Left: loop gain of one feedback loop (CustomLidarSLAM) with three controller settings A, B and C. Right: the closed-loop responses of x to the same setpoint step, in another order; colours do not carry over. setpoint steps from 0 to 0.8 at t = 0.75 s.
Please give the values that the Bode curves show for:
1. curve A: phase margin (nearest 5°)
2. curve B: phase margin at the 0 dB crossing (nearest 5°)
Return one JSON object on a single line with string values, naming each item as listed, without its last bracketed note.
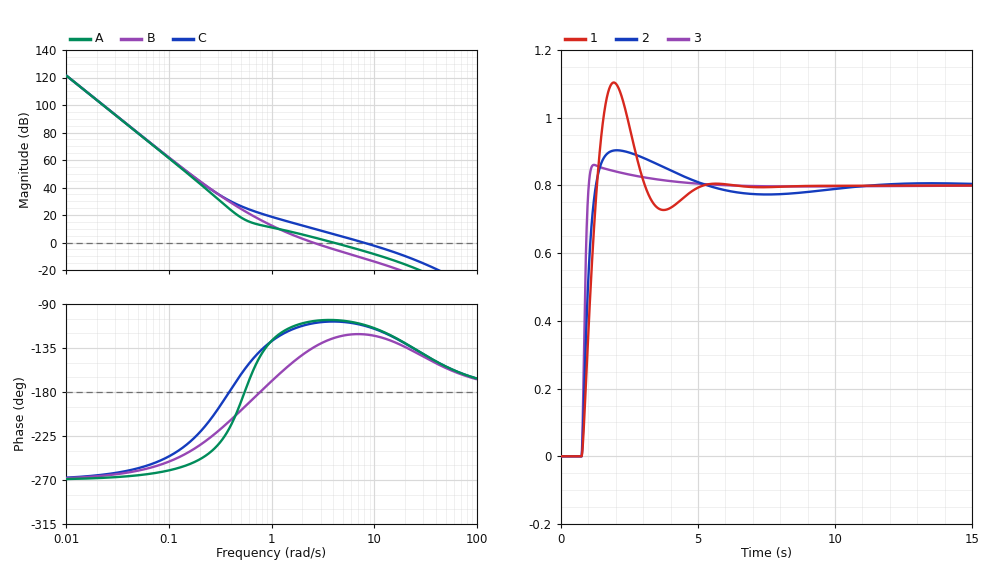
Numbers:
{"curve A: phase margin": "75°", "curve B: phase margin at the 0 dB crossing": "45°"}
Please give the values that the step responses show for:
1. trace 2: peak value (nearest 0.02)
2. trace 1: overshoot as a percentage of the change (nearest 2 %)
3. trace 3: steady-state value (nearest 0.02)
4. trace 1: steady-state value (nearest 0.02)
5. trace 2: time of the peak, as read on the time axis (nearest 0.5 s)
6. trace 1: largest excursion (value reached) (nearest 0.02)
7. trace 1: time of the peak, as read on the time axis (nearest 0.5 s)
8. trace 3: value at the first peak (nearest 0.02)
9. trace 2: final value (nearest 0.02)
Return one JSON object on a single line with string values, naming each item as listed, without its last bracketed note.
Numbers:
{"trace 2: peak value": "0.90", "trace 1: overshoot as a percentage of the change": "38 %", "trace 3: steady-state value": "0.80", "trace 1: steady-state value": "0.80", "trace 2: time of the peak, as read on the time axis": "2.0 s", "trace 1: largest excursion (value reached)": "1.10", "trace 1: time of the peak, as read on the time axis": "2.0 s", "trace 3: value at the first peak": "0.86", "trace 2: final value": "0.80"}
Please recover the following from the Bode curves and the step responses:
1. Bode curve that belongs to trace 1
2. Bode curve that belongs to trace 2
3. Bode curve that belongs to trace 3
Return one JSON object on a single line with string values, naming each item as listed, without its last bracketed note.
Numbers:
{"Bode curve that belongs to trace 1": "B", "Bode curve that belongs to trace 2": "A", "Bode curve that belongs to trace 3": "C"}
